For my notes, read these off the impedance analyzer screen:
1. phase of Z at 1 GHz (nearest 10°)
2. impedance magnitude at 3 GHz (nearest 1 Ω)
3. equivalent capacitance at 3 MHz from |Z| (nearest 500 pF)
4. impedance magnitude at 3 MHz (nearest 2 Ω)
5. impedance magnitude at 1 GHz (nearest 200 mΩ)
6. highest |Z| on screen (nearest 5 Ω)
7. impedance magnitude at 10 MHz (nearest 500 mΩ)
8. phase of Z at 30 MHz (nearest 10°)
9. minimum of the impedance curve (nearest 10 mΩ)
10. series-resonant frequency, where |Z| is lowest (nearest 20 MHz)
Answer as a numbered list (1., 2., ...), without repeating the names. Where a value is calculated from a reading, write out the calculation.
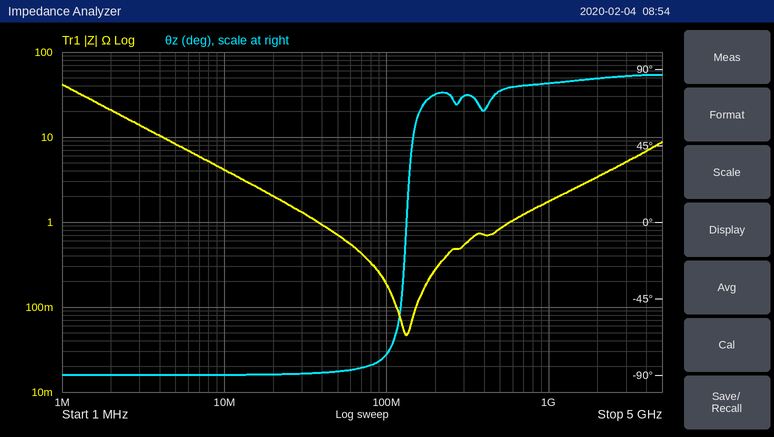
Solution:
1. 80°
2. 5 Ω
3. C = 1/(2π × 3 MHz × 14 Ω) ≈ 3.79 nF, so 4.0 nF to the nearest 500 pF
4. 14 Ω
5. 1.8 Ω
6. 40 Ω
7. 4.0 Ω
8. -90°
9. 50 mΩ
10. 140 MHz
